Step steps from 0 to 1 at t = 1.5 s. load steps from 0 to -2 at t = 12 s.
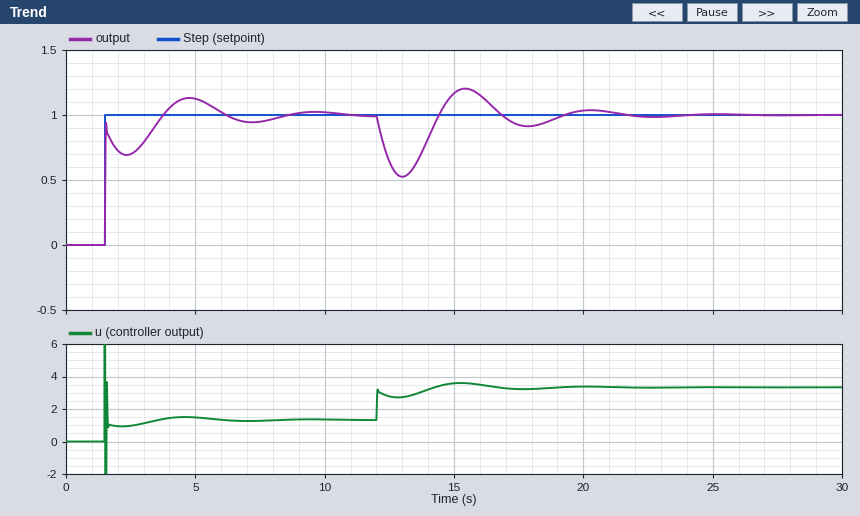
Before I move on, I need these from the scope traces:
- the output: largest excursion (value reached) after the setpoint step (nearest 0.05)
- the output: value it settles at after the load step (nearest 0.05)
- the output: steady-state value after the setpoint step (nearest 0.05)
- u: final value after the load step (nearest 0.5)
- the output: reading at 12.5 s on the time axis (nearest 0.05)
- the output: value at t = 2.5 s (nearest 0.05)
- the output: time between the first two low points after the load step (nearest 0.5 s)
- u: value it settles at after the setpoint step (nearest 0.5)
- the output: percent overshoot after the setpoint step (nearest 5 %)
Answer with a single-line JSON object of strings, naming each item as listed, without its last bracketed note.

{"the output: largest excursion (value reached) after the setpoint step": "1.15", "the output: value it settles at after the load step": "1.00", "the output: steady-state value after the setpoint step": "1.00", "u: final value after the load step": "3.5", "the output: reading at 12.5 s on the time axis": "0.65", "the output: value at t = 2.5 s": "0.70", "the output: time between the first two low points after the load step": "5.0 s", "u: value it settles at after the setpoint step": "1.5", "the output: percent overshoot after the setpoint step": "15 %"}
